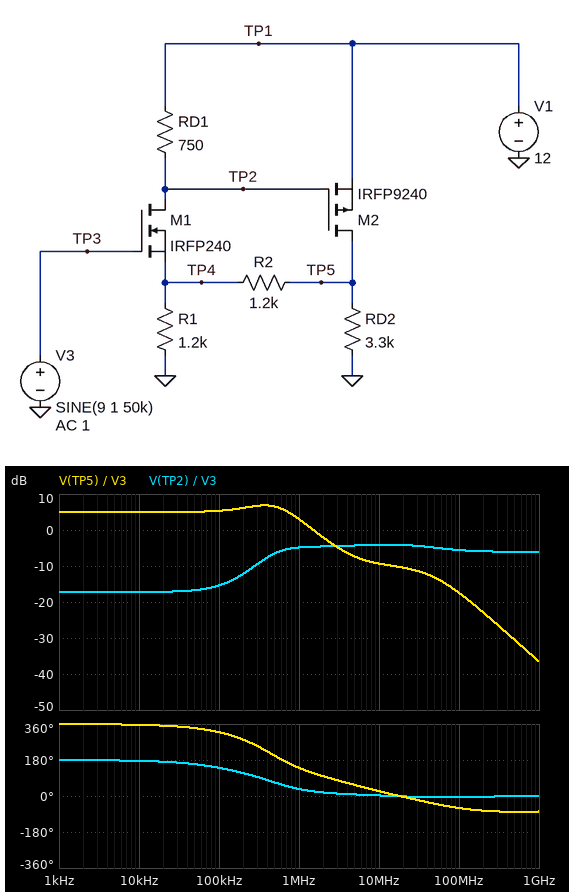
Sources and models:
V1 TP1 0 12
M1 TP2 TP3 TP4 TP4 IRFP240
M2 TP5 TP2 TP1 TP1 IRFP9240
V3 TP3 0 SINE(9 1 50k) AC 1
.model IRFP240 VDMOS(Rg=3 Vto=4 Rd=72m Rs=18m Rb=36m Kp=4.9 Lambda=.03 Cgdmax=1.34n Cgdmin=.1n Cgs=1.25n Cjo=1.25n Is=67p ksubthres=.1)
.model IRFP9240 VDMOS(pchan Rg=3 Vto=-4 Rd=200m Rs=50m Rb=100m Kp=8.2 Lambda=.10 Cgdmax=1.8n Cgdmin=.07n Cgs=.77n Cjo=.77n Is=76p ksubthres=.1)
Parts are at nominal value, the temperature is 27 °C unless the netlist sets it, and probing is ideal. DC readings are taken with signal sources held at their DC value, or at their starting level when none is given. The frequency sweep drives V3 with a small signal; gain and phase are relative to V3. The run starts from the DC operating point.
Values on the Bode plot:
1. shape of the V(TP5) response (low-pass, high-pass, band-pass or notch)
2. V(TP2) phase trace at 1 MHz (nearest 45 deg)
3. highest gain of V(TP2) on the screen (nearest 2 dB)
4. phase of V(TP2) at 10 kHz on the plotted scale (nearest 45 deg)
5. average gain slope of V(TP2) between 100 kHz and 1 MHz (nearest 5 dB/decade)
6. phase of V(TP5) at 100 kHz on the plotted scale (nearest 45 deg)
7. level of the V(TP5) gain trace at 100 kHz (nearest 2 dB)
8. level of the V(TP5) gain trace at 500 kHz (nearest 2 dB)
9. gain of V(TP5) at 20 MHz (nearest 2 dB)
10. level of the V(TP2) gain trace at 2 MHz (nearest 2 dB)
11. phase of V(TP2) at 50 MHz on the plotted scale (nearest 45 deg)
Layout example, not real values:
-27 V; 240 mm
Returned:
low-pass; 45 deg; -4 dB; 180 deg; 10 dB/decade; 315 deg; 6 dB; 6 dB; -10 dB; -4 dB; 0 deg
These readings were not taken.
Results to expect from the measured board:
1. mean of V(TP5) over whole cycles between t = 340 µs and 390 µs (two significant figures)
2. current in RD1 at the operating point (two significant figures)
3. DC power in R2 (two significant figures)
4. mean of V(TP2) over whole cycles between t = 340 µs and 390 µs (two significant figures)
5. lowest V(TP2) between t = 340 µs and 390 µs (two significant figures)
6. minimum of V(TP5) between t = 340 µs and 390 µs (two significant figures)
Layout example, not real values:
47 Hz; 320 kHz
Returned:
4.3 V; 5.0 mA; 740 µW; 8.4 V; 8.2 V; 3.0 V
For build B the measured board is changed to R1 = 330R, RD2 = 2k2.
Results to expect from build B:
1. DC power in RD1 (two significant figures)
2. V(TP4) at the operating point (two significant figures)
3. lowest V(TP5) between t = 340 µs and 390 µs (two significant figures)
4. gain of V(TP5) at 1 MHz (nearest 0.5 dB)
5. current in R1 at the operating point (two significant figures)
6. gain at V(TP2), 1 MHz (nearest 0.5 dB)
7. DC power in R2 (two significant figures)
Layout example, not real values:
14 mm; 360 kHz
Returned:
65 mW; 5.0 V; 12 V; -65.0 dB; 15 mA; -7.0 dB; 41 mW
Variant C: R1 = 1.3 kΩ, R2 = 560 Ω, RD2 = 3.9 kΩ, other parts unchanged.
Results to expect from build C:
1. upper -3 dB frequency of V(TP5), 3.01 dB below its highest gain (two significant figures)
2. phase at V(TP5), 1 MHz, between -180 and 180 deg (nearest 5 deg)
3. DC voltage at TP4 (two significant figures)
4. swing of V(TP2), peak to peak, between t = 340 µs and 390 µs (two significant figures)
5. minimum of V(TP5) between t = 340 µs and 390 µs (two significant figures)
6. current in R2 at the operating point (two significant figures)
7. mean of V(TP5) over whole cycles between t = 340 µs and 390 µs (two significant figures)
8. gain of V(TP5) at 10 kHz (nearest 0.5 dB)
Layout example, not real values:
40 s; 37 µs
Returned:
250 kHz; 45 deg; 5.1 V; 740 mV; 3.6 V; 1.0 mA; 4.6 V; 1.5 dB
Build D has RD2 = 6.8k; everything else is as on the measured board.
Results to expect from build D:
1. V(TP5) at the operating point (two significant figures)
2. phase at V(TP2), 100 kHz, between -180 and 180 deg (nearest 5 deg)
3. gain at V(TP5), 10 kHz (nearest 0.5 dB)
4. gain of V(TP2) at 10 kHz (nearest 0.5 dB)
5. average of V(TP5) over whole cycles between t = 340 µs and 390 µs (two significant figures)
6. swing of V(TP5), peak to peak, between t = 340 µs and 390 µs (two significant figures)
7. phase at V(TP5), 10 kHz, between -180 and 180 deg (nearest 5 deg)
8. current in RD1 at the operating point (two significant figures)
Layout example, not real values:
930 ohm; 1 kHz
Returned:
4.3 V; 115 deg; 1.5 dB; -6.0 dB; 4.6 V; 2.6 V; -5 deg; 4.8 mA
